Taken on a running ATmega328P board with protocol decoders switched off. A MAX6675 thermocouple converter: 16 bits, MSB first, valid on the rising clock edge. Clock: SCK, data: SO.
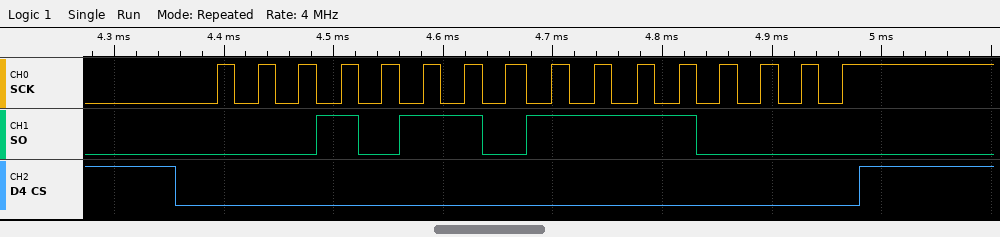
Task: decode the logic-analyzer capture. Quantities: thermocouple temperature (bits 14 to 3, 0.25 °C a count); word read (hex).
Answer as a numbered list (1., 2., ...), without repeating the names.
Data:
1. 183.50 °C
2. 0x16F0
